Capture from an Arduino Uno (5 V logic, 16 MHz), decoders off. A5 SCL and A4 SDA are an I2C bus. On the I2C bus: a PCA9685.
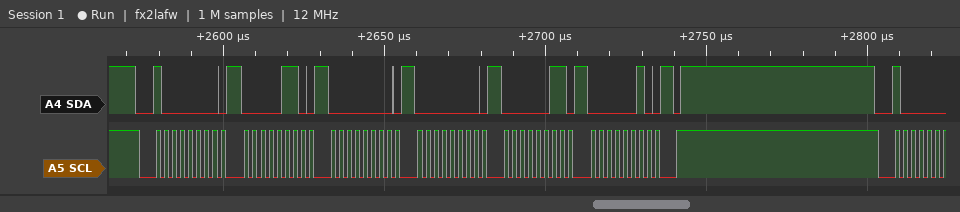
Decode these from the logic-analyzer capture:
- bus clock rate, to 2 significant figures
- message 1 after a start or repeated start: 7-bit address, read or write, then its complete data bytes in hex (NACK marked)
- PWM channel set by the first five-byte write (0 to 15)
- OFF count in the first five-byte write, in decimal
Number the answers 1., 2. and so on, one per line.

1. 400 kHz
2. 0x40 write: 06 00 00 03 02
3. 0
4. 515
